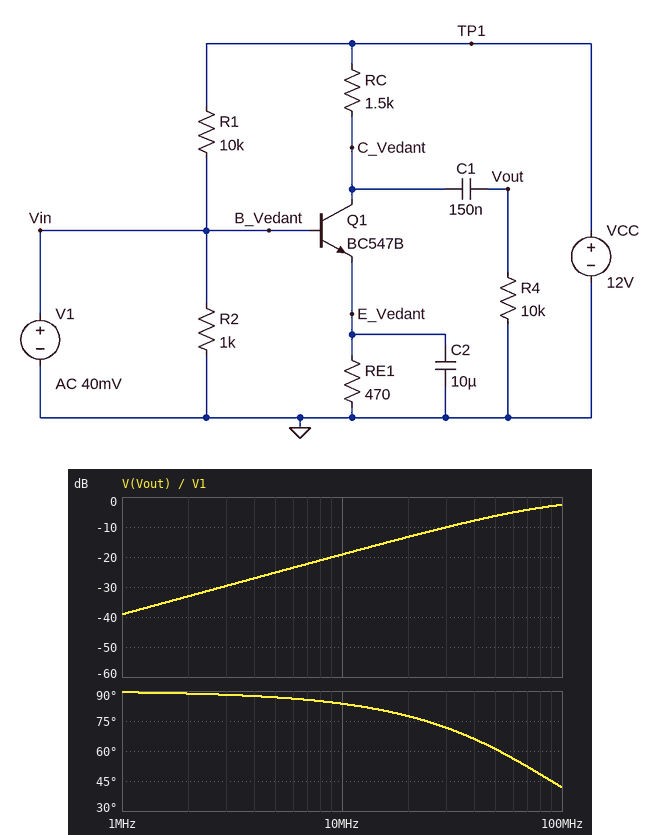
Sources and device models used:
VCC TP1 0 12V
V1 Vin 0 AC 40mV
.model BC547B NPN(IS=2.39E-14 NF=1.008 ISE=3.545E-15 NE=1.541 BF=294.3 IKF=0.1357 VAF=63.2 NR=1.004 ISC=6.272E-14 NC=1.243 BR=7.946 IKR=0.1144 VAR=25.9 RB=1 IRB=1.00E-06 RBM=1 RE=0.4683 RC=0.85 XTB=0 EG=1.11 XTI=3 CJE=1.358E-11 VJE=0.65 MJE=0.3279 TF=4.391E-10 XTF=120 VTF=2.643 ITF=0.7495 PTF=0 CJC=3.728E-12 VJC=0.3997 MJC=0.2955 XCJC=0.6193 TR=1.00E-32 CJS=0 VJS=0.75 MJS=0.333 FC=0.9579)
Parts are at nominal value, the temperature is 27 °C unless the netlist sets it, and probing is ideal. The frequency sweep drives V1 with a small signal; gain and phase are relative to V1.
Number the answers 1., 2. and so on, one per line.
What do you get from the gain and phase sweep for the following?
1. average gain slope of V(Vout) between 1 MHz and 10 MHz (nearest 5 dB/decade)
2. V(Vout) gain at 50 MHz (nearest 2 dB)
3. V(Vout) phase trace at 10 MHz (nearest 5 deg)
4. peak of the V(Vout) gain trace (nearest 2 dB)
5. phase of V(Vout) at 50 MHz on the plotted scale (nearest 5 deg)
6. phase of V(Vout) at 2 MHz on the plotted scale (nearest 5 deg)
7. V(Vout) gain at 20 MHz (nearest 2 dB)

1. 20 dB/decade
2. -6 dB
3. 85 deg
4. -2 dB
5. 60 deg
6. 90 deg
7. -14 dB
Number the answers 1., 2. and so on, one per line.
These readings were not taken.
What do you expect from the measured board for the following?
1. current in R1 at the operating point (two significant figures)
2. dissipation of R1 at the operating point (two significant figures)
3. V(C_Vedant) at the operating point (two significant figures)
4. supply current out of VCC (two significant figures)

1. 1.2 mA
2. 14 mW
3. 12 V
4. 1.2 mA
